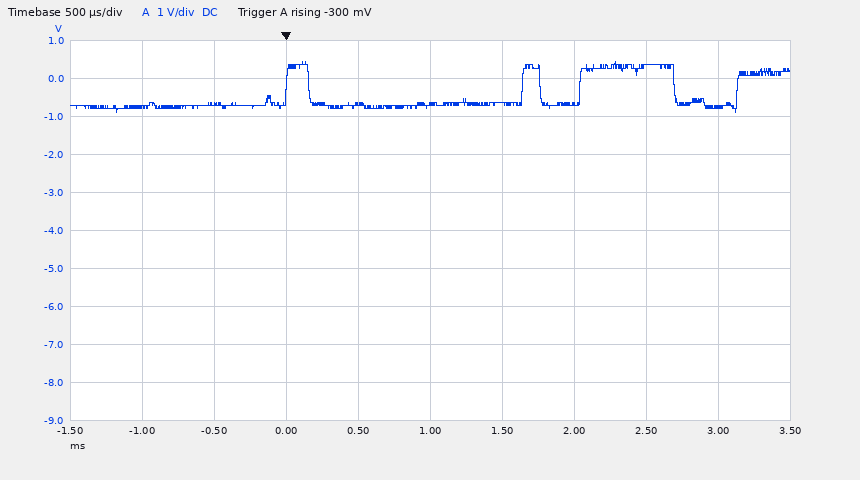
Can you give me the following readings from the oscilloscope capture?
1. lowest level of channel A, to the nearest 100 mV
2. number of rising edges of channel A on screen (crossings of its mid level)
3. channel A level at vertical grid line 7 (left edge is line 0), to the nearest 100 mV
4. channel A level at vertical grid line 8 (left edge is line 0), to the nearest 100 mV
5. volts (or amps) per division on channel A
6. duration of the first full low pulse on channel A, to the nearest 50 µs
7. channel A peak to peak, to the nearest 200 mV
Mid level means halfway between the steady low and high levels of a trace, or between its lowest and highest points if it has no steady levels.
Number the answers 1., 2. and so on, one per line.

1. -900 mV
2. 4
3. -700 mV
4. 300 mV
5. 1 V
6. 1.50 ms
7. 1.4 V
